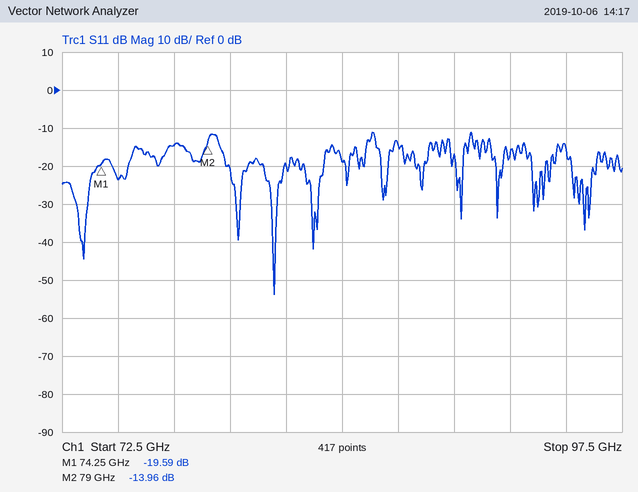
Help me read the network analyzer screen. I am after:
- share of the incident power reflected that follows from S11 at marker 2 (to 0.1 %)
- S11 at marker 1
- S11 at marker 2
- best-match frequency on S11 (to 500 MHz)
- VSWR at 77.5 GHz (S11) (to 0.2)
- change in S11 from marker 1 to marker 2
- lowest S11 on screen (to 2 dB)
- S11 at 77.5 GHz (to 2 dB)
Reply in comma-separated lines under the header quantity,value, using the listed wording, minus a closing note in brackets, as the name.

quantity,value
share of the incident power reflected that follows from S11 at marker 2,4.0 %
S11 at marker 1,-19.59 dB
S11 at marker 2,-13.96 dB
best-match frequency on S11,82.0 GHz
VSWR at 77.5 GHz (S11),1.4
change in S11 from marker 1 to marker 2,5.63 dB
lowest S11 on screen,-54 dB
S11 at 77.5 GHz,-14 dB
